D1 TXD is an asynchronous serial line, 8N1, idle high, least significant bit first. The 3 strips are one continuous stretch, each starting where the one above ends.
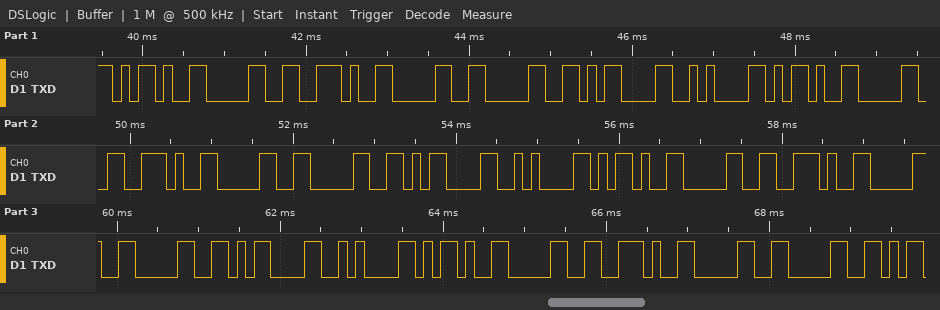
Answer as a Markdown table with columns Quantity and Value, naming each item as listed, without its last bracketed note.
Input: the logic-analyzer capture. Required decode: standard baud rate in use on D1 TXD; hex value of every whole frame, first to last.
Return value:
| Quantity | Value |
|---|---|
| standard baud rate in use on D1 TXD | 9600 baud |
| hex value of every whole frame, first to last | 2D 30 2E 30 30 0D 0A 2D 30 2E 30 30 0D 0A 2D 30 2E 30 30 0D 0A 2D 30 2E 30 30 |
